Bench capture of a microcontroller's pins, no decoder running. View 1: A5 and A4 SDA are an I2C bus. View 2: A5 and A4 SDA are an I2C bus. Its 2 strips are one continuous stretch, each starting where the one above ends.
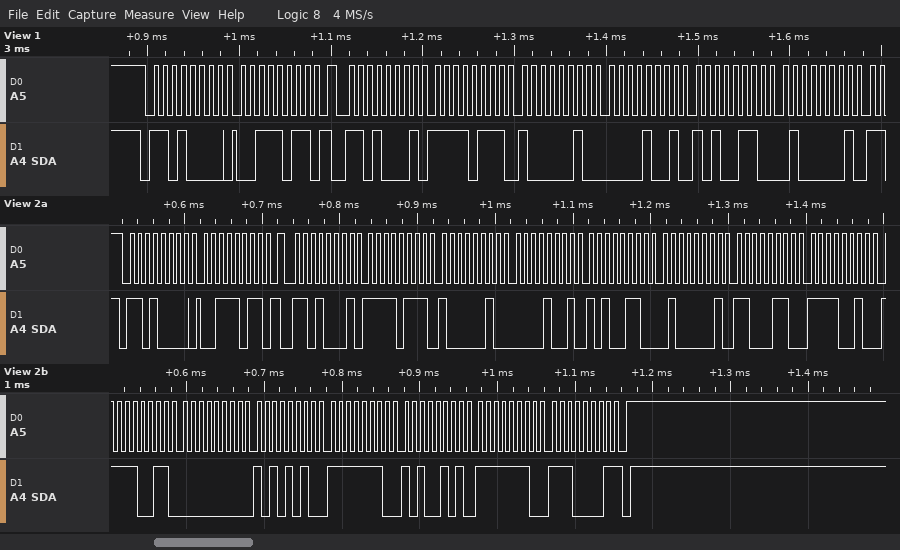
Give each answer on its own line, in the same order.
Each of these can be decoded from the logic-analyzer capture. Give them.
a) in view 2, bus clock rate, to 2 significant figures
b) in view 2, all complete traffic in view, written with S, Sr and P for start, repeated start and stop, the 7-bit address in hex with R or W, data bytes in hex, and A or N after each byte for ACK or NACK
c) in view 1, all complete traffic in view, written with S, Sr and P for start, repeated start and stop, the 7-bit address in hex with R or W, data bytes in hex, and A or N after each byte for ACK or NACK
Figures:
100 kHz
S 68W A 3B A Sr 68R A F7 A 82 A 09 A A6 A 41 A C6 A F2 A F3 A 00 A AA A FE A A5 A FE A E1 N P
S 68W A 3B A Sr 68R A F7 A 82 A 09 A A6 A 41 A
